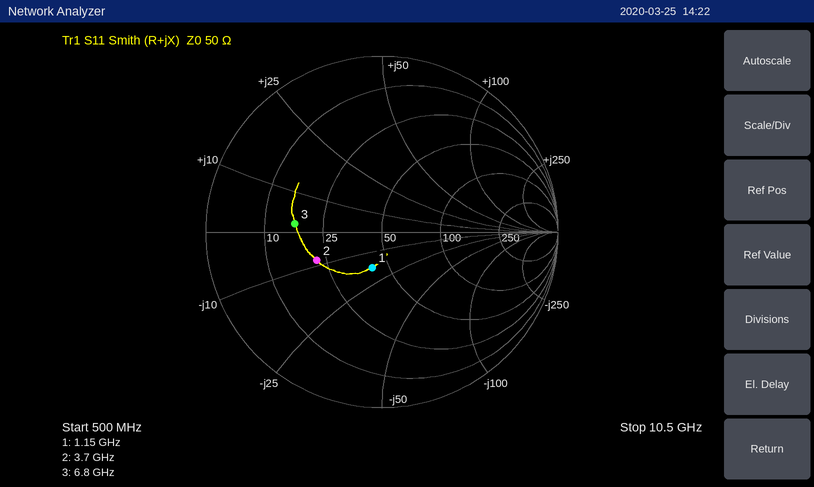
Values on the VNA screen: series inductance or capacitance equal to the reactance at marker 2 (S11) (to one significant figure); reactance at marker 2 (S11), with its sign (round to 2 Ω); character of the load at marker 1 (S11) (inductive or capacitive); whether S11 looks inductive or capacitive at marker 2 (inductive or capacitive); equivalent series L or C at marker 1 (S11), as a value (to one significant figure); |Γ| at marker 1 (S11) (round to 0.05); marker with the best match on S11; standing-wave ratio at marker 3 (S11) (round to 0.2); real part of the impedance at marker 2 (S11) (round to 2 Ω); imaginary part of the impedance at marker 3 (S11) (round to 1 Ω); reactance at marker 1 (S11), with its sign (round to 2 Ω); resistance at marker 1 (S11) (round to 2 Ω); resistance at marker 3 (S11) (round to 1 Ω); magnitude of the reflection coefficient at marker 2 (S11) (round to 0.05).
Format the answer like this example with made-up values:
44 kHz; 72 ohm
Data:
5 pF; -8 Ω; capacitive; capacitive; 8 pF; 0.20; marker 1; 3.0; 22 Ω; +2 Ω; -18 Ω; 42 Ω; 17 Ω; 0.40
